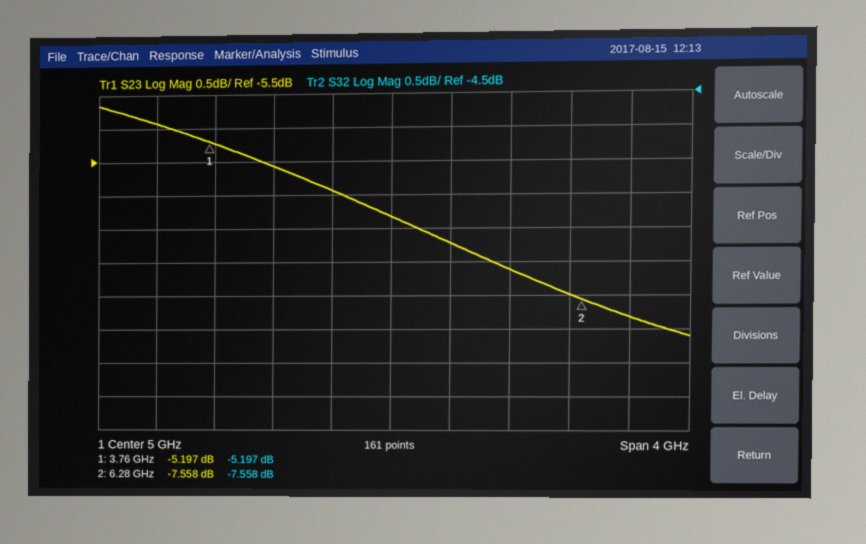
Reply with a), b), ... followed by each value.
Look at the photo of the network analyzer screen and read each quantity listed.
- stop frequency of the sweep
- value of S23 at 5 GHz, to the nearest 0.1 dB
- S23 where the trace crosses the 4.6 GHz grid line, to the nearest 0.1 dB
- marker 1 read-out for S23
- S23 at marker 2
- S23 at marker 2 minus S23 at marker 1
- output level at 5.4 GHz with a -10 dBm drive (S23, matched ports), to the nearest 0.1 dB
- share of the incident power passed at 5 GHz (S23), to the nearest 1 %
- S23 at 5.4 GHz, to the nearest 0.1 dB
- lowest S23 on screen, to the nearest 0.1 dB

a) 7 GHz
b) -6.3 dB
c) -5.9 dB
d) -5.197 dB
e) -7.558 dB
f) -2.361 dB
g) -16.7 dBm
h) 23 %
i) -6.7 dB
j) -8.1 dB
